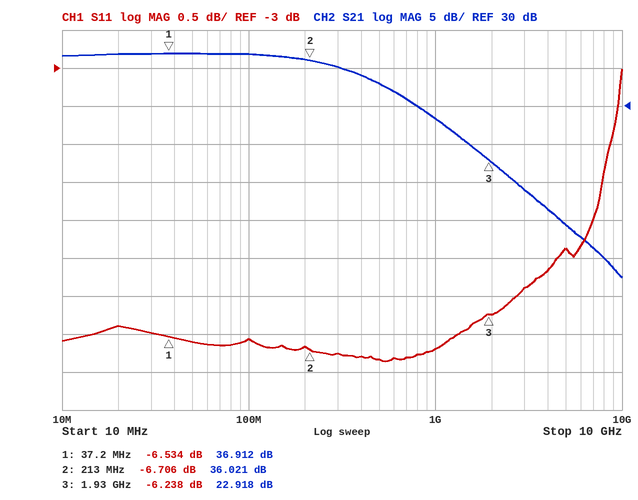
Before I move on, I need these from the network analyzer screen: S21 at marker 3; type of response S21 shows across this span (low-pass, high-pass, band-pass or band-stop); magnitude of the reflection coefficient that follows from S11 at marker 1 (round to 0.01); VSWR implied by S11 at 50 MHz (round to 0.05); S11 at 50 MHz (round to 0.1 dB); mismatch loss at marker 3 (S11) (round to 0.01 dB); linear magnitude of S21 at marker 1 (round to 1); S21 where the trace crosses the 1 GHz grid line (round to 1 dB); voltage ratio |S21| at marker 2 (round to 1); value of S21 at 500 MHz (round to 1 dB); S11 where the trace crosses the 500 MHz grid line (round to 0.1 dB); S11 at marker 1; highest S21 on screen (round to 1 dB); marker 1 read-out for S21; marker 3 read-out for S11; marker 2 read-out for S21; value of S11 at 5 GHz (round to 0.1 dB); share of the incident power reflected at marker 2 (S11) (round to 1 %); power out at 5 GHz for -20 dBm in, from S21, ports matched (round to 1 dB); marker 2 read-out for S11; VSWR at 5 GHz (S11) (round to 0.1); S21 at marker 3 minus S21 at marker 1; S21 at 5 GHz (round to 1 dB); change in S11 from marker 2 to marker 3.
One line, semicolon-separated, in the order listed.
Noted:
22.918 dB; low-pass; 0.47; 2.75; -6.6 dB; 1.18 dB; 70; 28 dB; 63; 33 dB; -6.8 dB; -6.534 dB; 37 dB; 36.912 dB; -6.238 dB; 36.021 dB; -5.4 dB; 21 %; -6 dBm; -6.706 dB; 3.3; -13.994 dB; 14 dB; 0.468 dB
